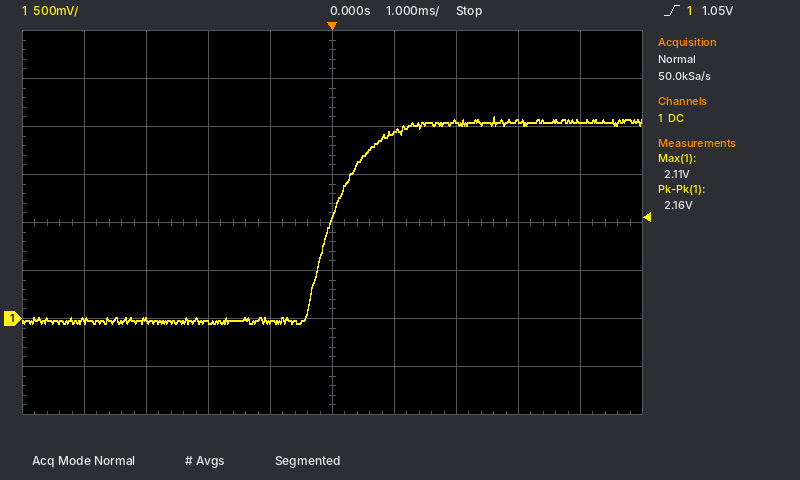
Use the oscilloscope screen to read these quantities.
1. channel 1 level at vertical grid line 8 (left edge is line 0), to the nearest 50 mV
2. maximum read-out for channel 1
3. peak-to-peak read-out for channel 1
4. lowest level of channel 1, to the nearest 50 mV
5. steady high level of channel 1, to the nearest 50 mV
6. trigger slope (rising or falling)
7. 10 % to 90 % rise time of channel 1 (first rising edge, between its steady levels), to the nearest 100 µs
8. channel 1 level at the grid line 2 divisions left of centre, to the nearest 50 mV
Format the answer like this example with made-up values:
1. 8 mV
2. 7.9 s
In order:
1. 2.05 V
2. 2.11 V
3. 2.16 V
4. -50 mV
5. 2.05 V
6. rising
7. 1.1 ms
8. -50 mV
